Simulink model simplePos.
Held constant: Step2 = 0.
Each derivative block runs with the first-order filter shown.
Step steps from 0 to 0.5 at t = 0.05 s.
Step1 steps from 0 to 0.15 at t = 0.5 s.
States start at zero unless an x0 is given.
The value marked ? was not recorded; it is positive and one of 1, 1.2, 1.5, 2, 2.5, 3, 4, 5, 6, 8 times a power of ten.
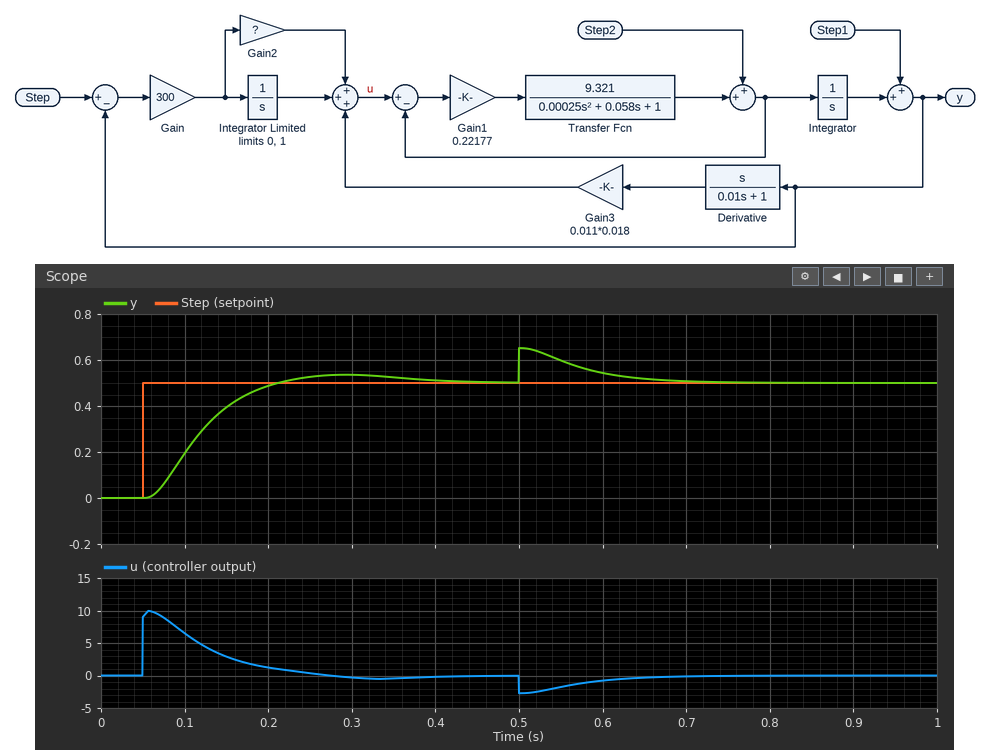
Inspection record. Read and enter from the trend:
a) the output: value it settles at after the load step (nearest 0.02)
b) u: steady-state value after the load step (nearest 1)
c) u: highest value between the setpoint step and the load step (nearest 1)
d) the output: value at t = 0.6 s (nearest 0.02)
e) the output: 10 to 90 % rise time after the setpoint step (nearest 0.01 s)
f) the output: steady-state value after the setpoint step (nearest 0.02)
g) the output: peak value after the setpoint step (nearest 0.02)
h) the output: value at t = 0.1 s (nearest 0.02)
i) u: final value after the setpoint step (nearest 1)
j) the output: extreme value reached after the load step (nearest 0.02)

0.50
0
10
0.54
0.10 s
0.50
0.54
0.20
0
0.66
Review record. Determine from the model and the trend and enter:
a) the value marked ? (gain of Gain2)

0.06
